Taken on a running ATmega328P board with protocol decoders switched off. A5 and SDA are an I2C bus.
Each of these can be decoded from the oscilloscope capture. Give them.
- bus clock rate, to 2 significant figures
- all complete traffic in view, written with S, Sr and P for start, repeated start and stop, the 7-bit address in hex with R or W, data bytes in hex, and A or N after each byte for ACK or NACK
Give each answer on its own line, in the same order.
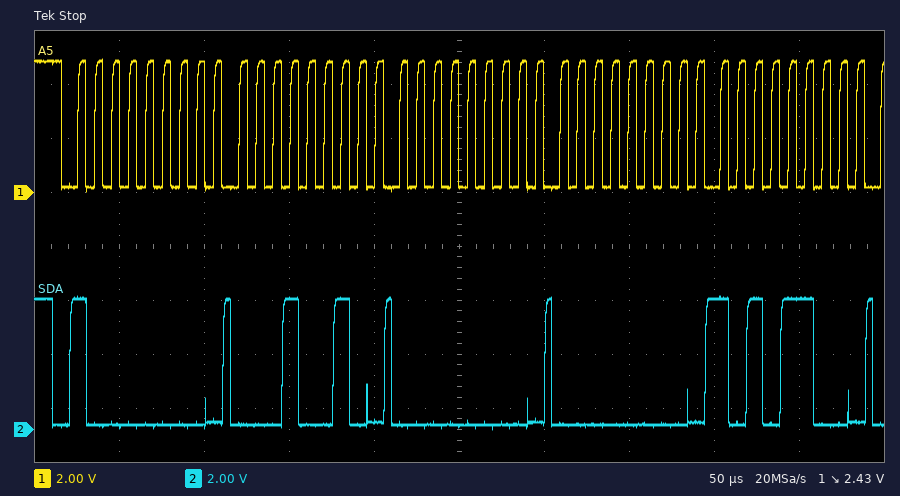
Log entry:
100 kHz
S 40W A 12 A 00 A 00 A AC A
